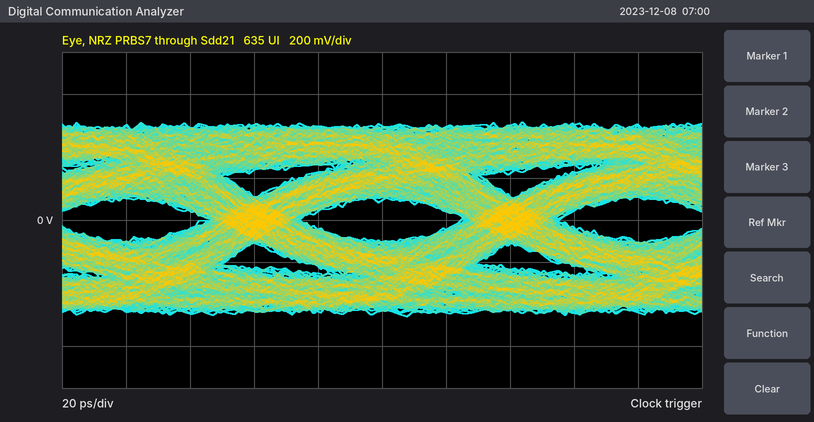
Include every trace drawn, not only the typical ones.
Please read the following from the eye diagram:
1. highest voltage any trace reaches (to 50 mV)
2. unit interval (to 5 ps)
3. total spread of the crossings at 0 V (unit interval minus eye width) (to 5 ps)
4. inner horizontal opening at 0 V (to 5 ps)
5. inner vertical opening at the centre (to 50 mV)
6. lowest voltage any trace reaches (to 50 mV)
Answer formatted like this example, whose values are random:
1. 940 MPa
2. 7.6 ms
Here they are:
1. 450 mV
2. 80 ps
3. 30 ps
4. 50 ps
5. 200 mV
6. -450 mV
